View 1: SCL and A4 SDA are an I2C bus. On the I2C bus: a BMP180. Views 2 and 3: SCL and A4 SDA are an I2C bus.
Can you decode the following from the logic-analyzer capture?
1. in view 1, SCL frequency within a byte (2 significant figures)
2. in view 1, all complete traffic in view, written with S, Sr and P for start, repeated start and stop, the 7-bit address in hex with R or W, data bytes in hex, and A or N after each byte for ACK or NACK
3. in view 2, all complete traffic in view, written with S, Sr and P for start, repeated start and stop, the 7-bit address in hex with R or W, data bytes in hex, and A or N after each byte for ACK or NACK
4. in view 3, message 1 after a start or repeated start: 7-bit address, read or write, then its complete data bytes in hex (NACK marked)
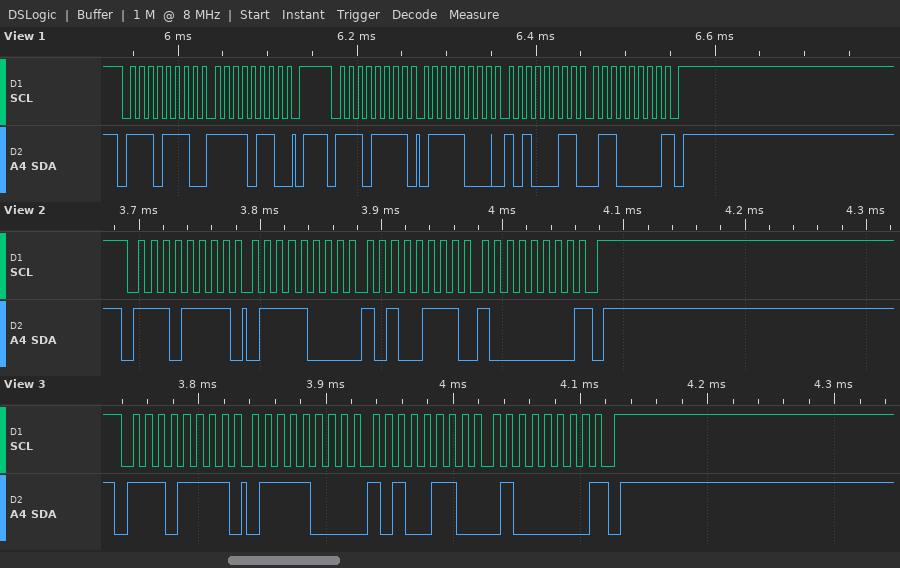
100 kHz
S 77W A F6 A P S 77R A 78 A A3 A 60 N P
S 77R A 78 A A7 A 80 N P
0x77 read: 78 A6 40 NACK
